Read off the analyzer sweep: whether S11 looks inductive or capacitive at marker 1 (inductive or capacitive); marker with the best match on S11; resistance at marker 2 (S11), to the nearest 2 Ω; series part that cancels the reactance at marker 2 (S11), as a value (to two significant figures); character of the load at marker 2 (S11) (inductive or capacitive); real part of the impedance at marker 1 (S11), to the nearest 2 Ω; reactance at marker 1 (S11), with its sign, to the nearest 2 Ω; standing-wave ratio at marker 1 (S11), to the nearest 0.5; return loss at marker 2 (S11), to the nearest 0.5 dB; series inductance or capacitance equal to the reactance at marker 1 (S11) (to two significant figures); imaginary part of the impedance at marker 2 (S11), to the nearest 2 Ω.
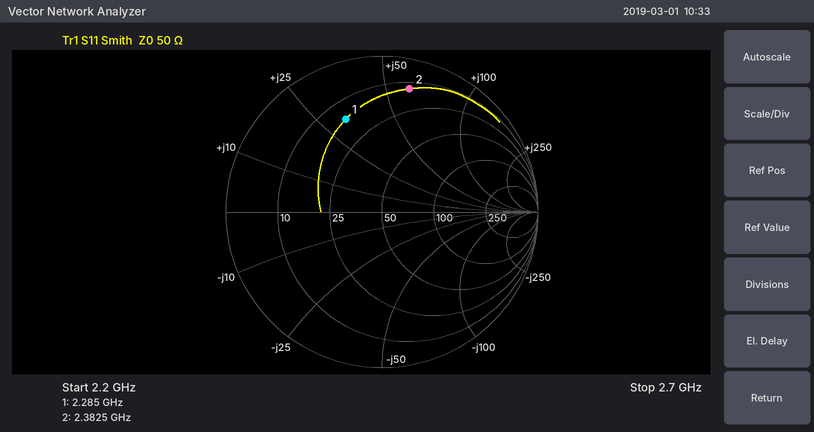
inductive
marker 1
14 Ω
1.1 pF
inductive
16 Ω
+32 Ω
4.5
2.0 dB
2.2 nH
+60 Ω
